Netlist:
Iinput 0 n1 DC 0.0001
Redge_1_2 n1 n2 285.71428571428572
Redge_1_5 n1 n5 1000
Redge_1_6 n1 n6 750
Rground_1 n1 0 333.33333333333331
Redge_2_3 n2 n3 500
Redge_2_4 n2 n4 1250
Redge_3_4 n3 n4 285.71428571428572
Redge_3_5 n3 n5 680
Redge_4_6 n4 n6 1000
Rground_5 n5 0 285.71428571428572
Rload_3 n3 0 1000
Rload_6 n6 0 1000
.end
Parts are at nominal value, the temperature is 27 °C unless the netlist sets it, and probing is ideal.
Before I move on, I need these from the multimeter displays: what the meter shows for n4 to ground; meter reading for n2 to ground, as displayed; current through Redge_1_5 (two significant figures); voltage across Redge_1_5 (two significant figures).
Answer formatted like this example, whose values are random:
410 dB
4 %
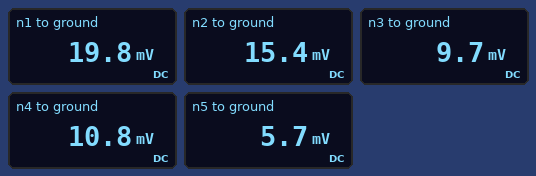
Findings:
10.8 mV
15.4 mV
14 µA
14 mV
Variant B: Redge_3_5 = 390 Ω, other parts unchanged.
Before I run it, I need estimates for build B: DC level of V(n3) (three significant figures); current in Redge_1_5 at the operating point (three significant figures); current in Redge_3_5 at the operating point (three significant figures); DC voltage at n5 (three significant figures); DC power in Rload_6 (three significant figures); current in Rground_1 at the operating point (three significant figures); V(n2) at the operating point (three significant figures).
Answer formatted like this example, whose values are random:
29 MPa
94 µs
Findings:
9.01 mV
13.6 µA
7.59 µA
6.05 mV
120 nW
58.9 µA
15.1 mV
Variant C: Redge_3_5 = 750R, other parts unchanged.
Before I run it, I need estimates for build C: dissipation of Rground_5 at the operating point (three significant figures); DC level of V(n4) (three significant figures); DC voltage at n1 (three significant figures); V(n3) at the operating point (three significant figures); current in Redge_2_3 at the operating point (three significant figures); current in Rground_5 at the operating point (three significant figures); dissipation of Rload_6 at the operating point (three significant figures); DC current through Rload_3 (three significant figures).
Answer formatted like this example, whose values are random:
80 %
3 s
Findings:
111 nW
10.9 mV
19.8 mV
9.78 mV
11.4 µA
19.7 µA
125 nW
9.78 µA
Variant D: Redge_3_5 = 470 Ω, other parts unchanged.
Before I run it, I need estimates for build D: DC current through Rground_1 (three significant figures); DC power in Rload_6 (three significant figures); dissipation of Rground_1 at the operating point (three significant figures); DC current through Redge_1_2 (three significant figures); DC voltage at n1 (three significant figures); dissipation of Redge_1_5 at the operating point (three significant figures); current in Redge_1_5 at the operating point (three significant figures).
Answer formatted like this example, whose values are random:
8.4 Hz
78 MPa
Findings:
59.0 µA
121 nW
1.16 µW
15.7 µA
19.7 mV
189 nW
13.7 µA
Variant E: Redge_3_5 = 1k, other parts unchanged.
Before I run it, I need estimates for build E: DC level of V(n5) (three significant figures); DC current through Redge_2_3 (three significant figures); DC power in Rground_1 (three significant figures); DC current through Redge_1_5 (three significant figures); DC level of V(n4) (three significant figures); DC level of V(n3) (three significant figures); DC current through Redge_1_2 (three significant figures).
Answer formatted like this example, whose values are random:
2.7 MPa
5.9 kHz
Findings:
5.45 mV
11.1 µA
1.18 µW
14.4 µA
11.2 mV
10.1 mV
14.7 µA
